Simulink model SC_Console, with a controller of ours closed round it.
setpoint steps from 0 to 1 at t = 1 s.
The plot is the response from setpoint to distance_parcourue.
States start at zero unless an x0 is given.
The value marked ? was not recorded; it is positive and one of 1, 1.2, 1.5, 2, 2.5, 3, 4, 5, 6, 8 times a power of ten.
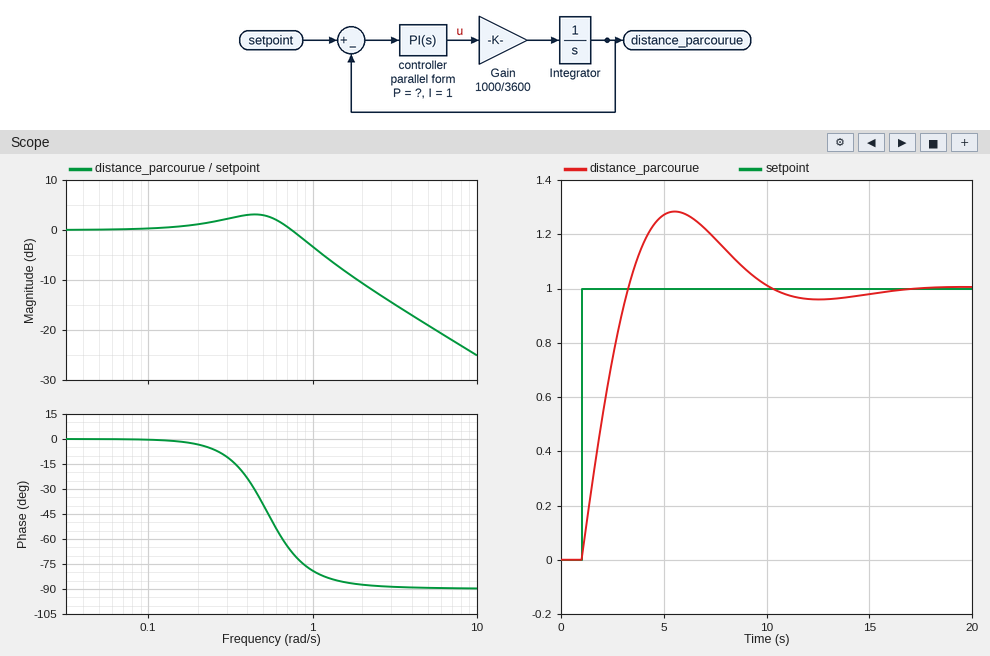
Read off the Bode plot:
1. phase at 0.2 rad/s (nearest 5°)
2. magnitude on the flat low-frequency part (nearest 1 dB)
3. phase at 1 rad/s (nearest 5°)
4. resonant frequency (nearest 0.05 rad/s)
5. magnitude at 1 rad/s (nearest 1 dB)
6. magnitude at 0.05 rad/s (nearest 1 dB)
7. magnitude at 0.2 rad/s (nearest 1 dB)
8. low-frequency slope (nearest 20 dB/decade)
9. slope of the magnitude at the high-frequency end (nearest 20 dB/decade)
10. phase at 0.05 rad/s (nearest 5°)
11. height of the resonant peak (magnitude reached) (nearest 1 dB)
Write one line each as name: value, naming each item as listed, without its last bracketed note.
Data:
phase at 0.2 rad/s: -5°
magnitude on the flat low-frequency part: 0 dB
phase at 1 rad/s: -80°
resonant frequency: 0.45 rad/s
magnitude at 1 rad/s: -3 dB
magnitude at 0.05 rad/s: 0 dB
magnitude at 0.2 rad/s: 1 dB
low-frequency slope: 0 dB/decade
slope of the magnitude at the high-frequency end: -20 dB/decade
phase at 0.05 rad/s: 0°
height of the resonant peak (magnitude reached): 3 dB
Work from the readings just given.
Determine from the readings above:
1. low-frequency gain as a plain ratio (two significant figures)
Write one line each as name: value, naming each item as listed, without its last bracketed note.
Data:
low-frequency gain as a plain ratio: 1.0
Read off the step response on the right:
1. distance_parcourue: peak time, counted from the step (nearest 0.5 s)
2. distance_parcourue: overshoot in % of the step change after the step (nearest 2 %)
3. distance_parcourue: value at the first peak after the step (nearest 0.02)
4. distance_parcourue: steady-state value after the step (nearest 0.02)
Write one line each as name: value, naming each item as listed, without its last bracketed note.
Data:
distance_parcourue: peak time, counted from the step: 4.5 s
distance_parcourue: overshoot in % of the step change after the step: 28 %
distance_parcourue: value at the first peak after the step: 1.28
distance_parcourue: steady-state value after the step: 1.00
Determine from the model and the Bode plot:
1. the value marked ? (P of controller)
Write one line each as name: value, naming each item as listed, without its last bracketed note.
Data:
the value marked ?: 2
